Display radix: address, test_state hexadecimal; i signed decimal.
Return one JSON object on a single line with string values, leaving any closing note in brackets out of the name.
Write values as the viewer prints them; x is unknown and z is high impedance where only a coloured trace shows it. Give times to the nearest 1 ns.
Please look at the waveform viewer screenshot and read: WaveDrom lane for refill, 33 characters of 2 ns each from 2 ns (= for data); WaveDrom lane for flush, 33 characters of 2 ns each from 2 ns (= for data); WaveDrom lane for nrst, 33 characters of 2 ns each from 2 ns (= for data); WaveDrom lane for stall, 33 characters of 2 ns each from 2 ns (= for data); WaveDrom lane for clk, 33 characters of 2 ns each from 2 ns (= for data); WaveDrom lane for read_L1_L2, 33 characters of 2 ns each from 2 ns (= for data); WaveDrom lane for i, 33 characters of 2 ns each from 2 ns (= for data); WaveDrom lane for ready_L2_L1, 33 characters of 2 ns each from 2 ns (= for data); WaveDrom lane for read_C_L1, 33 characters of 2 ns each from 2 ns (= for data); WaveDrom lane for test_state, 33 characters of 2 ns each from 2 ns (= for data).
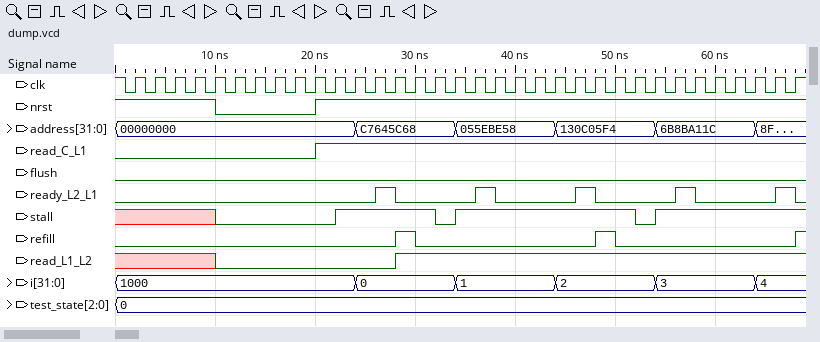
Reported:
{"WaveDrom lane for refill, 33 characters of 2 ns each from 2 ns": "{name: 'refill', wave: '0............10........10........'}", "WaveDrom lane for flush, 33 characters of 2 ns each from 2 ns": "{name: 'flush', wave: '0................................'}", "WaveDrom lane for nrst, 33 characters of 2 ns each from 2 ns": "{name: 'nrst', wave: '1...0....1.......................'}", "WaveDrom lane for stall, 33 characters of 2 ns each from 2 ns": "{name: 'stall', wave: 'x...0.....1....01........01......'}", "WaveDrom lane for clk, 33 characters of 2 ns each from 2 ns": "{name: 'clk', wave: 'p................................'}", "WaveDrom lane for read_L1_L2, 33 characters of 2 ns each from 2 ns": "{name: 'read_L1_L2', wave: 'x...0........1...................'}", "WaveDrom lane for i, 33 characters of 2 ns each from 2 ns": "{name: 'i', wave: '=..........=....=....=....=....=.', data: '1000 0 1 2 3 4'}", "WaveDrom lane for ready_L2_L1, 33 characters of 2 ns each from 2 ns": "{name: 'ready_L2_L1', wave: '0...........10...10...10...10...1'}", "WaveDrom lane for read_C_L1, 33 characters of 2 ns each from 2 ns": "{name: 'read_C_L1', wave: '0........1.......................'}", "WaveDrom lane for test_state, 33 characters of 2 ns each from 2 ns": "{name: 'test_state', wave: '=................................', data: '0'}"}
